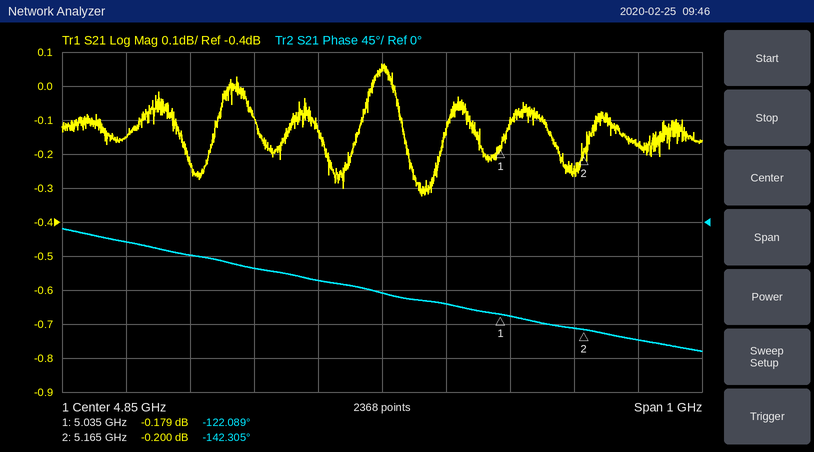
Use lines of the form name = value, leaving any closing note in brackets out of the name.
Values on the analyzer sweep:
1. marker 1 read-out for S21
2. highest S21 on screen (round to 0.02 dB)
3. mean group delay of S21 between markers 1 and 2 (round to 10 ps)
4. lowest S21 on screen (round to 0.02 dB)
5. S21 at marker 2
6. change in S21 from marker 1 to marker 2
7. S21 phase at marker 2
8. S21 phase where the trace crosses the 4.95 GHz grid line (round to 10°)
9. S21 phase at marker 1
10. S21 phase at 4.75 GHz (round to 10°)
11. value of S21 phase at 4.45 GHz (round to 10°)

marker 1 read-out for S21 = -0.179 dB
highest S21 on screen = 0.06 dB
mean group delay of S21 between markers 1 and 2 = 430 ps
lowest S21 on screen = -0.32 dB
S21 at marker 2 = -0.200 dB
change in S21 from marker 1 to marker 2 = -0.021 dB
S21 phase at marker 2 = -142.305°
S21 phase where the trace crosses the 4.95 GHz grid line = -110°
S21 phase at marker 1 = -122.089°
S21 phase at 4.75 GHz = -80°
value of S21 phase at 4.45 GHz = -30°
